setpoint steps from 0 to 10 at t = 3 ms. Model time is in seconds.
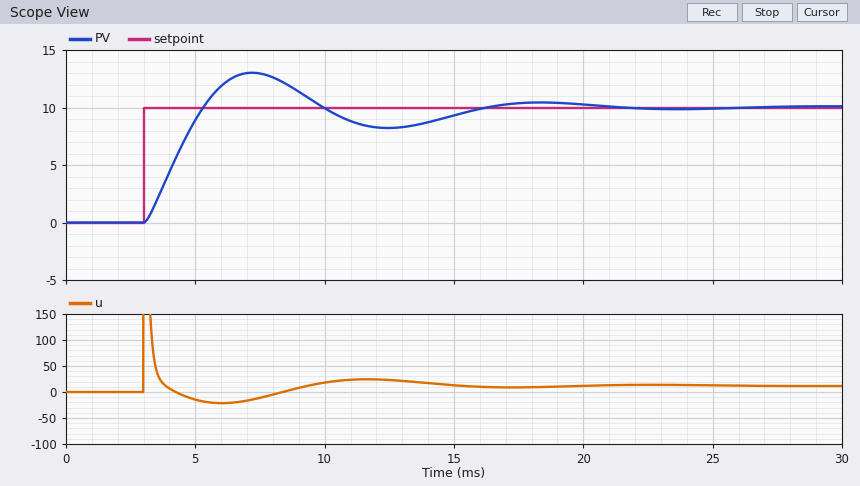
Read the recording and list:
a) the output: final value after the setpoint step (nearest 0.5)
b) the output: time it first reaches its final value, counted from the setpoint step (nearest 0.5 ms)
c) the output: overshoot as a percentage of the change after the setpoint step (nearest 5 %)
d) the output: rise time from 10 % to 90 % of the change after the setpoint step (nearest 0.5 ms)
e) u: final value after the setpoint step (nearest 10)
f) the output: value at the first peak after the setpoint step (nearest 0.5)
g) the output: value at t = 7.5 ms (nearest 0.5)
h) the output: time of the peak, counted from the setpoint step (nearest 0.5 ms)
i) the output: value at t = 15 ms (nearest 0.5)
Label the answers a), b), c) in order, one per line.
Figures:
a) 10.0
b) 2.5 ms
c) 30 %
d) 1.5 ms
e) 10
f) 13.0
g) 13.0
h) 4.0 ms
i) 9.5
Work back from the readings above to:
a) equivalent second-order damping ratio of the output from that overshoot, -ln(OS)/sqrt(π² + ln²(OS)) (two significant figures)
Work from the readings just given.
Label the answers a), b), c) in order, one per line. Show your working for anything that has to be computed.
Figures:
a) ln(0.3) = -1.204; 1.204 / sqrt(9.870 + 1.450) = 0.36
